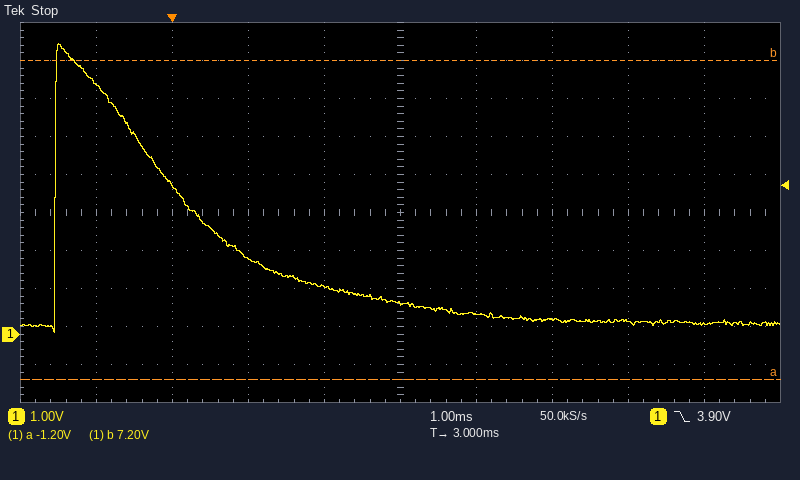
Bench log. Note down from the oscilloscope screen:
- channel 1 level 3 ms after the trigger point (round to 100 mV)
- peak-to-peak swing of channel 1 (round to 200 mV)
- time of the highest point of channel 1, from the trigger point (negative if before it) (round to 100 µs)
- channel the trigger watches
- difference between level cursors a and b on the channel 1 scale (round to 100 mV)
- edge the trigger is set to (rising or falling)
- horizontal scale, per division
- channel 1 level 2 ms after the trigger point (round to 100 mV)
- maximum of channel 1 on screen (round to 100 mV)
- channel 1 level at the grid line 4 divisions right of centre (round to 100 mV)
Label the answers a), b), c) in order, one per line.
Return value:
a) 800 mV
b) 7.6 V
c) -1.5 ms
d) channel 1
e) 8.4 V
f) falling
g) 1 ms
h) 1.3 V
i) 7.6 V
j) 300 mV
